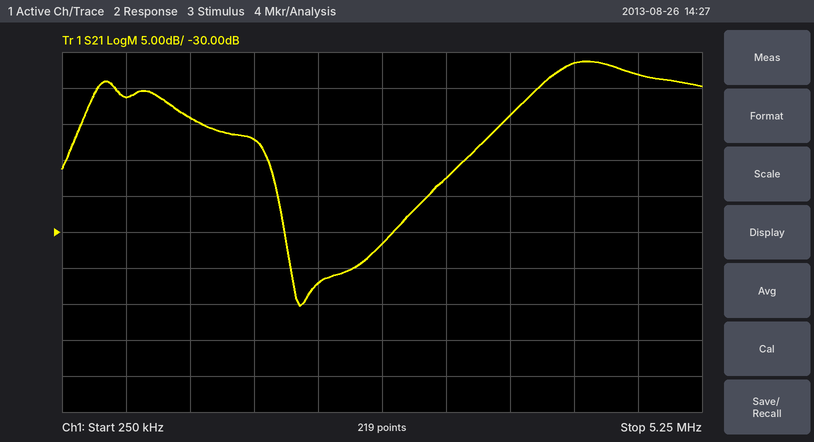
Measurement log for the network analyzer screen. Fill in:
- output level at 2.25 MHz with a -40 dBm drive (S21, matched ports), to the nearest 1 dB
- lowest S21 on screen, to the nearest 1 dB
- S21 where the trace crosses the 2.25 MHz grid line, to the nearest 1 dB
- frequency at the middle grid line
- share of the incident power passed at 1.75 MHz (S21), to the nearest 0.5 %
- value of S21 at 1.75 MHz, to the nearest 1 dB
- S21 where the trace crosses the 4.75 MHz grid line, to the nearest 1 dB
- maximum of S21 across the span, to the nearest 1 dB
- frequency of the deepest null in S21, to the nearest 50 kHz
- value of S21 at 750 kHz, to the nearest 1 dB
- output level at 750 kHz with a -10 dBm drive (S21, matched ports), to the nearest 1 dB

-77 dBm
-40 dB
-37 dB
2.75 MHz
2.0 %
-17 dB
-8 dB
-6 dB
2.10 MHz
-11 dB
-21 dBm
